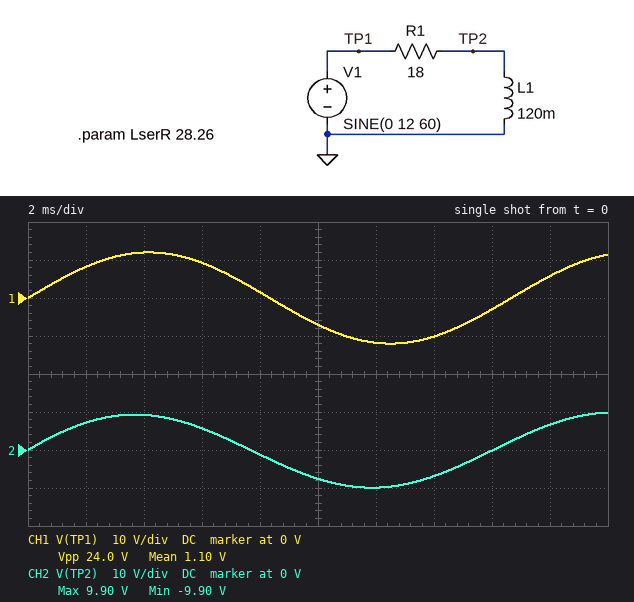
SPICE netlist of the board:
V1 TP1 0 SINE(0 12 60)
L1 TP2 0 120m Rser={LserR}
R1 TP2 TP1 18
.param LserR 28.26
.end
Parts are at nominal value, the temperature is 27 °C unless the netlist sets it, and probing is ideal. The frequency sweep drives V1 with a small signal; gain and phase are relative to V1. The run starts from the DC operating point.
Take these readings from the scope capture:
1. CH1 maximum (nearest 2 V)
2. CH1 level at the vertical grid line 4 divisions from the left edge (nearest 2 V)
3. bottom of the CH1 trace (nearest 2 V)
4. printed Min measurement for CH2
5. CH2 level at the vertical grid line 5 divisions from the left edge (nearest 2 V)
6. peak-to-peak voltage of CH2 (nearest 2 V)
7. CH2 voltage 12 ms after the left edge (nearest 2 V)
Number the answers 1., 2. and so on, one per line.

1. 12 V
2. 2 V
3. -12 V
4. -9.90 V
5. -8 V
6. 20 V
7. -10 V
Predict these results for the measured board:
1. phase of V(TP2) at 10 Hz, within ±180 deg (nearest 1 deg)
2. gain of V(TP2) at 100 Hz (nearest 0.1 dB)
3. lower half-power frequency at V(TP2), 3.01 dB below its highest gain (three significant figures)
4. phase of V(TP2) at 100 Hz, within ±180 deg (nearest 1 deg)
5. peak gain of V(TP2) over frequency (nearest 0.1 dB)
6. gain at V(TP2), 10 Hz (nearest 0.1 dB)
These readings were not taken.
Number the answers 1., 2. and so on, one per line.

1. 6 deg
2. -0.8 dB
3. 30.9 Hz
4. 11 deg
5. 0 dB
6. -4.1 dB
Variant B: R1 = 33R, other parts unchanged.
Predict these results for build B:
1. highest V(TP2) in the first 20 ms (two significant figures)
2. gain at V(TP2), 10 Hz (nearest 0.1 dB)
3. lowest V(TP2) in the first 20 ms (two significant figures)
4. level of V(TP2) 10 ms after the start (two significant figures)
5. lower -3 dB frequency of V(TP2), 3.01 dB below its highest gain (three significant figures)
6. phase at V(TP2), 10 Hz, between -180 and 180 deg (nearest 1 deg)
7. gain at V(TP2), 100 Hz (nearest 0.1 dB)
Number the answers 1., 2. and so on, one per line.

1. 8.4 V
2. -6.5 dB
3. -8.4 V
4. -7.1 V
5. 61.6 Hz
6. 8 deg
7. -1.6 dB
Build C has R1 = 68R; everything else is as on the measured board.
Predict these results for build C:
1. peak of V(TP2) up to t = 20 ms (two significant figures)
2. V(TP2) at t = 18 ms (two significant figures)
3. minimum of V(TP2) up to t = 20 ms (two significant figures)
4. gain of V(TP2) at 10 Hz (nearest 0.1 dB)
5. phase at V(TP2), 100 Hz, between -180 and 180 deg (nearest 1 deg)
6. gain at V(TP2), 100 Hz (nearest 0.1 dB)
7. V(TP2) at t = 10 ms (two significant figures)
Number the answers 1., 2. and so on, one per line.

1. 6.0 V
2. 5.3 V
3. -6.0 V
4. -10.4 dB
5. 31 deg
6. -3.6 dB
7. -5.6 V
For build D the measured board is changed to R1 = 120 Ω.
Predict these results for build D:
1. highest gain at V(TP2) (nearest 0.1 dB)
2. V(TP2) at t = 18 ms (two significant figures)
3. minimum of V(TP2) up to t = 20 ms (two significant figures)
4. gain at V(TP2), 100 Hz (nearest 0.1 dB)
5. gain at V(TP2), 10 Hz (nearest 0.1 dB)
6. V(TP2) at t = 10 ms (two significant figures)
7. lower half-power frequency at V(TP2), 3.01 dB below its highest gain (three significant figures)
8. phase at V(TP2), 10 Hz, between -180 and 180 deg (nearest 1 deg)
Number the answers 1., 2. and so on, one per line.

1. 0 dB
2. 3.9 V
3. -4.1 V
4. -6.3 dB
5. -14.1 dB
6. -4.0 V
7. 189 Hz
8. 12 deg
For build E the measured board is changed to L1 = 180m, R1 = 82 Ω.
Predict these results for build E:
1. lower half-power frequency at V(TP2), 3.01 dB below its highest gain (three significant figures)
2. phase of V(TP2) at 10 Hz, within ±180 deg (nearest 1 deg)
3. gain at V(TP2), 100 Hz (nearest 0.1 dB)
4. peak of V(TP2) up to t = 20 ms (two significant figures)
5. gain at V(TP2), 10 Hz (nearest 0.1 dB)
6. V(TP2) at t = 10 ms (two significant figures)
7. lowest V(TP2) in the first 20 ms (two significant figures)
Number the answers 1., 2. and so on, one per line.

1. 90.9 Hz
2. 16 deg
3. -2.6 dB
4. 6.8 V
5. -11.2 dB
6. -6.5 V
7. -6.8 V
